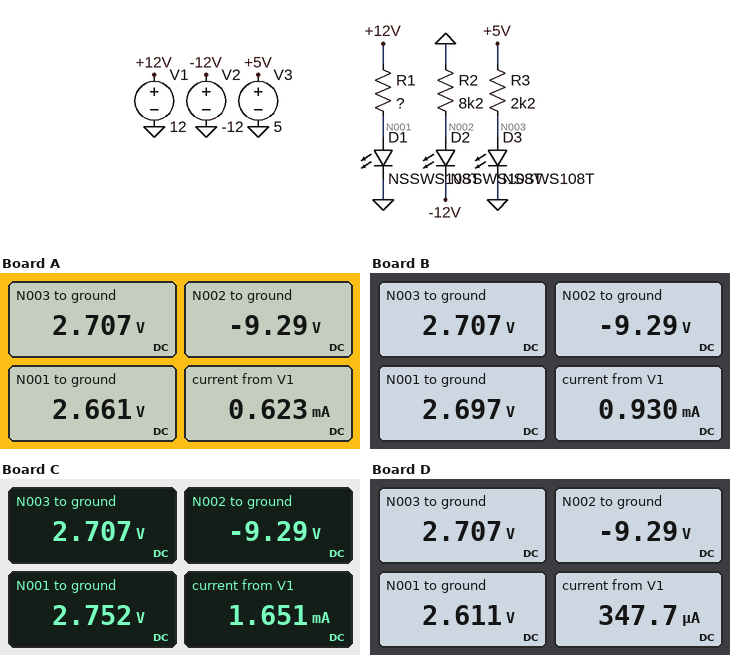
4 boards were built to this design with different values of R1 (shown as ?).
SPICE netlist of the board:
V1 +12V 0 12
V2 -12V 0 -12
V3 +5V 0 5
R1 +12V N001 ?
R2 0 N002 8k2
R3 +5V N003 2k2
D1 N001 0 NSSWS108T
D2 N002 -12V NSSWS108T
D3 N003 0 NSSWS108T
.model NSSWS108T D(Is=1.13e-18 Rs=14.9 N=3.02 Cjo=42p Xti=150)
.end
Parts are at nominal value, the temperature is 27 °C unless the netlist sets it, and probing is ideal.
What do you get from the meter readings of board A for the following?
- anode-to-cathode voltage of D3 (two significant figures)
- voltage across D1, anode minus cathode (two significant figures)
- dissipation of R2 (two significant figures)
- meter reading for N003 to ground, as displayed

2.7 V
2.7 V
11 mW
2.707 V
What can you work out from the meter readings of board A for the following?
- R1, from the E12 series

15 kΩ
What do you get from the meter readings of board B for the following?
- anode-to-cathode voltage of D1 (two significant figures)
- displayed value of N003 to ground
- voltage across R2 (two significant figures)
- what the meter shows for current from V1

2.7 V
2.707 V
9.3 V
0.930 mA
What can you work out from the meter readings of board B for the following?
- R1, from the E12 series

10 kΩ
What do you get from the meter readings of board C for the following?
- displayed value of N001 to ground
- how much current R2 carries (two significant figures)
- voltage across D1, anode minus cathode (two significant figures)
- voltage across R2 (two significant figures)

2.752 V
1.1 mA
2.8 V
9.3 V
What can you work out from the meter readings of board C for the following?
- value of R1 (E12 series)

5.6 kΩ
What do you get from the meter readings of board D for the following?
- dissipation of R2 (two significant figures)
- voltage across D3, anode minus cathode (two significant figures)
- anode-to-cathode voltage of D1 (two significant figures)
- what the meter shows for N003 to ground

11 mW
2.7 V
2.6 V
2.707 V
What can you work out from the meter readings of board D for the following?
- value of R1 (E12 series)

27 kΩ
